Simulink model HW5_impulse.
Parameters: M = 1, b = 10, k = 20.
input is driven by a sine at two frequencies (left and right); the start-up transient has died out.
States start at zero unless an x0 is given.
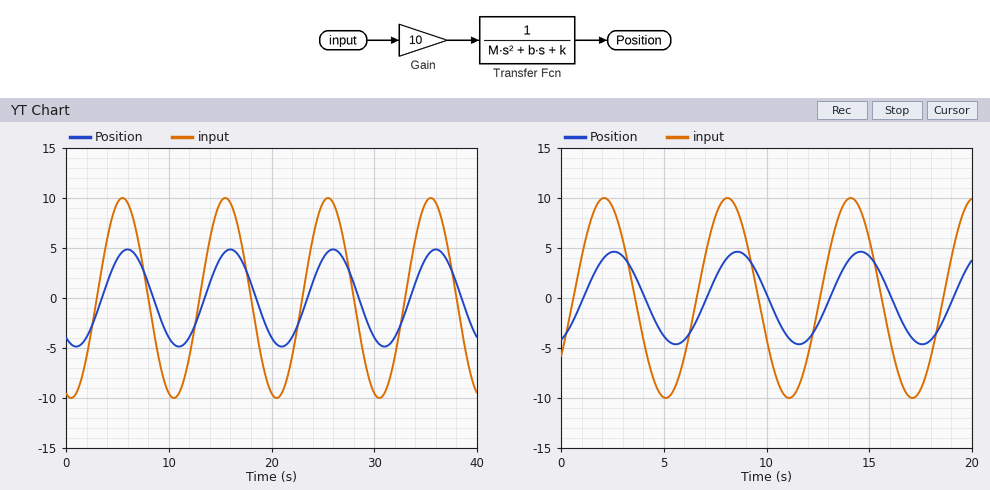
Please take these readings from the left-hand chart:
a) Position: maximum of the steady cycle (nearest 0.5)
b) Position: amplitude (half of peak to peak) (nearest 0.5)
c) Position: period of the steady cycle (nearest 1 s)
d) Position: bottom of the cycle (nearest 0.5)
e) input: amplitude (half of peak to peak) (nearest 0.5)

5.0
5.0
10 s
-5.0
10.0
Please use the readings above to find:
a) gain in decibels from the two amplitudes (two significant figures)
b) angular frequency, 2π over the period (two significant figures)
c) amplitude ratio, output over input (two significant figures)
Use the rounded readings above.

-6.0 dB
0.63 rad/s
0.50
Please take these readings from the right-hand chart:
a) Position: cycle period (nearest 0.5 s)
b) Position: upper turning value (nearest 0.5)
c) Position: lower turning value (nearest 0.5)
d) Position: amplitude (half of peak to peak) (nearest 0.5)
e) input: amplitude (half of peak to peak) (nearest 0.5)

6.0 s
4.5
-4.5
4.5
10.0
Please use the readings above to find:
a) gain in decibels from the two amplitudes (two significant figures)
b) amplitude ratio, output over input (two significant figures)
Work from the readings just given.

-6.9 dB
0.45
